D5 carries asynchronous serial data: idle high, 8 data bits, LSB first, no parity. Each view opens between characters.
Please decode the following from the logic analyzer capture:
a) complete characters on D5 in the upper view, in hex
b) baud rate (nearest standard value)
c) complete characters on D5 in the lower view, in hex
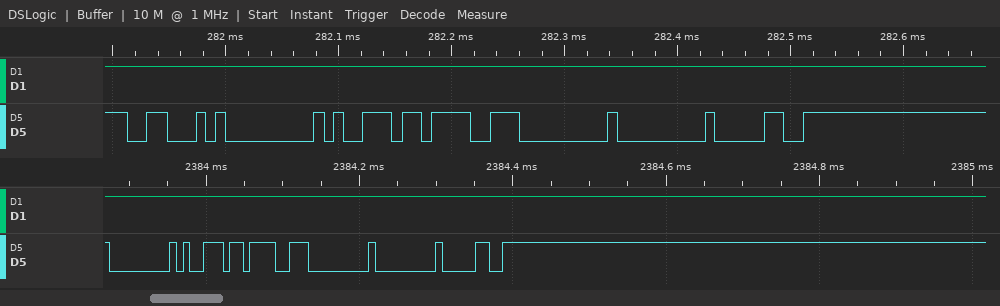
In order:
46, 00, B9, CF, 00, 00, 30
115200 baud
00, B9, CF, 00, 00, 30
